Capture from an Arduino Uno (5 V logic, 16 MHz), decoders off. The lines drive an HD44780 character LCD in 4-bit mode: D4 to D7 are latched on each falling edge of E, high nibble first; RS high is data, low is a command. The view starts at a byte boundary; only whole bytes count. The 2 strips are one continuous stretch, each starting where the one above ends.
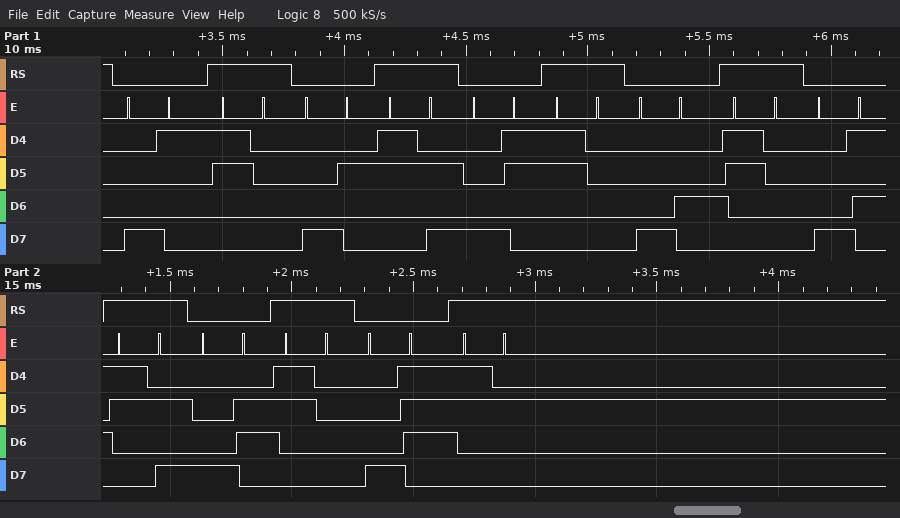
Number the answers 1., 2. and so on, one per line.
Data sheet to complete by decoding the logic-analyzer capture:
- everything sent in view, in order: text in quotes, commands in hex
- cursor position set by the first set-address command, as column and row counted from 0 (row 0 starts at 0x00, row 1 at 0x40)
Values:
1. 0x81 "0" 0x82 ":" 0x83 "0" 0x84 "0" 0x85 ":" 0x86 "0" 0x87 "2"
2. column 1, row 0
